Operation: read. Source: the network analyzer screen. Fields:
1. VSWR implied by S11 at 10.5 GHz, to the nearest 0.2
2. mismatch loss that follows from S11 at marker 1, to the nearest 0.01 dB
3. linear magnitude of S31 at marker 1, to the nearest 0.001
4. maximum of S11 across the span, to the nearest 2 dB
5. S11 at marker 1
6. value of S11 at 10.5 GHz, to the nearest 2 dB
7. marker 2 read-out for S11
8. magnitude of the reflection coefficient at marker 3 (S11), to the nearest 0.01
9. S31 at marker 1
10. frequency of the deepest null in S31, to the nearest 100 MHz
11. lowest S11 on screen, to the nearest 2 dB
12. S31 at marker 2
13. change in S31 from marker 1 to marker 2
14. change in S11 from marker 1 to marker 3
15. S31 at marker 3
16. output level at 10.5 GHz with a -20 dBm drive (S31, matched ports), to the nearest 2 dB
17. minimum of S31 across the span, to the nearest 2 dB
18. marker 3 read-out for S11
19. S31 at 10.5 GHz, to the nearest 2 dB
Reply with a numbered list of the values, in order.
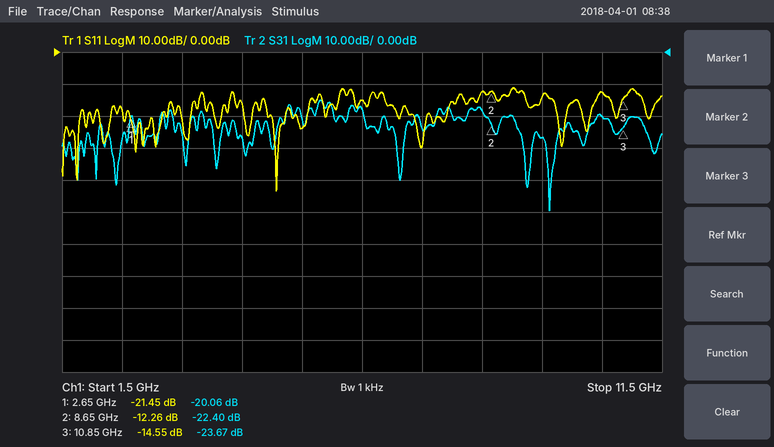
1. 1.6
2. 0.03 dB
3. 0.099
4. -12 dB
5. -21.45 dB
6. -12 dB
7. -12.26 dB
8. 0.19
9. -20.06 dB
10. 9.6 GHz
11. -44 dB
12. -22.40 dB
13. -2.34 dB
14. 6.90 dB
15. -23.67 dB
16. -40 dBm
17. -50 dB
18. -14.55 dB
19. -20 dB
